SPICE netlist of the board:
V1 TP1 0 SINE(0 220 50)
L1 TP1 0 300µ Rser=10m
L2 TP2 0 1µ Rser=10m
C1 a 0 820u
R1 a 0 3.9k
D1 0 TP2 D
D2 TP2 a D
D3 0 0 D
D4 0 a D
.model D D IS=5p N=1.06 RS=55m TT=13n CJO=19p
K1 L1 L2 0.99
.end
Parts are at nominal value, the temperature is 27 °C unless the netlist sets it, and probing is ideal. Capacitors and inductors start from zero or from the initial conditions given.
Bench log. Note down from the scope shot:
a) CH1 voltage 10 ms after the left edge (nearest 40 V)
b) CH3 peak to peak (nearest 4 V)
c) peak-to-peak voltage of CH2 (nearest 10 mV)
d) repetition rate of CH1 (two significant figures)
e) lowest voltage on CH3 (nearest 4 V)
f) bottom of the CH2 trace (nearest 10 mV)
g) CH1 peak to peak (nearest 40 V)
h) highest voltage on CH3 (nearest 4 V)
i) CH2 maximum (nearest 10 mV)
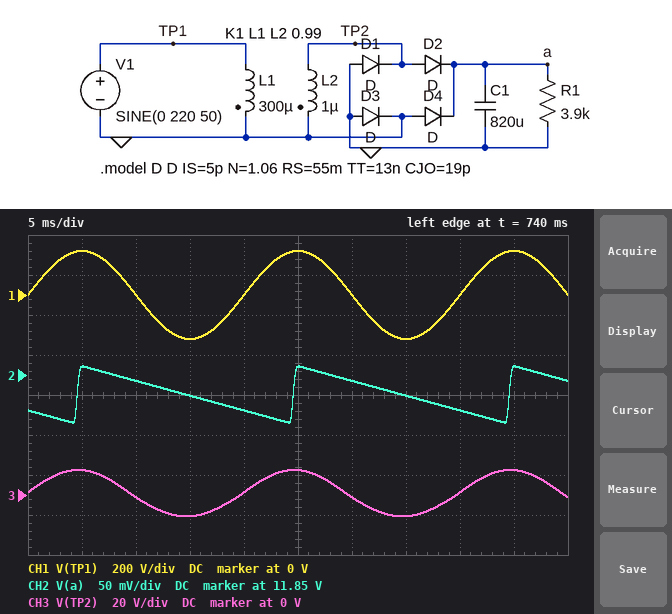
0 V
24 V
70 mV
50 Hz
-12 V
11.79 V
440 V
12 V
11.86 V
